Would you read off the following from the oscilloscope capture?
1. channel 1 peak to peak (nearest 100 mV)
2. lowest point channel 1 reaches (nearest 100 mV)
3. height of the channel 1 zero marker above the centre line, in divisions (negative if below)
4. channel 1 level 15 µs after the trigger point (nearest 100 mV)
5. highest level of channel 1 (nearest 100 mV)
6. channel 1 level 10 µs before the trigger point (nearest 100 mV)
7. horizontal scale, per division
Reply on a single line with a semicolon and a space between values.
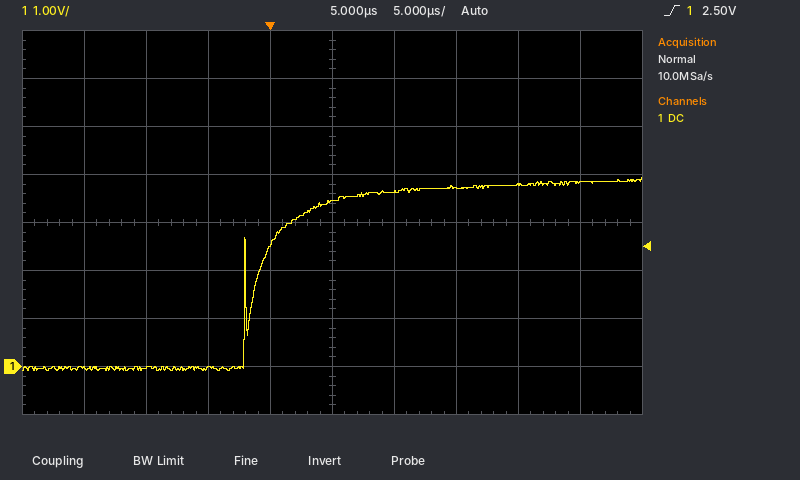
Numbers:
4.0 V; -100 mV; -3.0 div; 3.7 V; 3.9 V; 0.0 V; 5 µs
